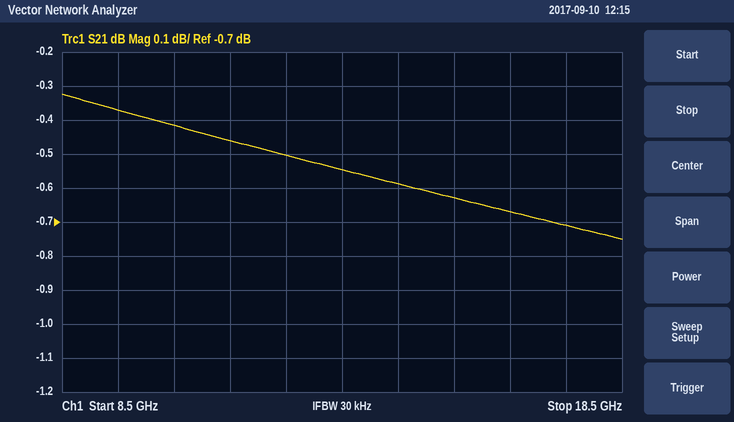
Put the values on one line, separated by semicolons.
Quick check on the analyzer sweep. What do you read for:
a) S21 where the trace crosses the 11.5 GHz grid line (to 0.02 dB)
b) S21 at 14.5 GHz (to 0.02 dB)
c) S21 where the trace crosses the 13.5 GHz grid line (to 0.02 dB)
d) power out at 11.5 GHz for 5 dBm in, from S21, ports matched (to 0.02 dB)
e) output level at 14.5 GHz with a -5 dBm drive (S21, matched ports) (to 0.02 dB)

-0.46 dB; -0.58 dB; -0.54 dB; 4.54 dBm; -5.58 dBm
